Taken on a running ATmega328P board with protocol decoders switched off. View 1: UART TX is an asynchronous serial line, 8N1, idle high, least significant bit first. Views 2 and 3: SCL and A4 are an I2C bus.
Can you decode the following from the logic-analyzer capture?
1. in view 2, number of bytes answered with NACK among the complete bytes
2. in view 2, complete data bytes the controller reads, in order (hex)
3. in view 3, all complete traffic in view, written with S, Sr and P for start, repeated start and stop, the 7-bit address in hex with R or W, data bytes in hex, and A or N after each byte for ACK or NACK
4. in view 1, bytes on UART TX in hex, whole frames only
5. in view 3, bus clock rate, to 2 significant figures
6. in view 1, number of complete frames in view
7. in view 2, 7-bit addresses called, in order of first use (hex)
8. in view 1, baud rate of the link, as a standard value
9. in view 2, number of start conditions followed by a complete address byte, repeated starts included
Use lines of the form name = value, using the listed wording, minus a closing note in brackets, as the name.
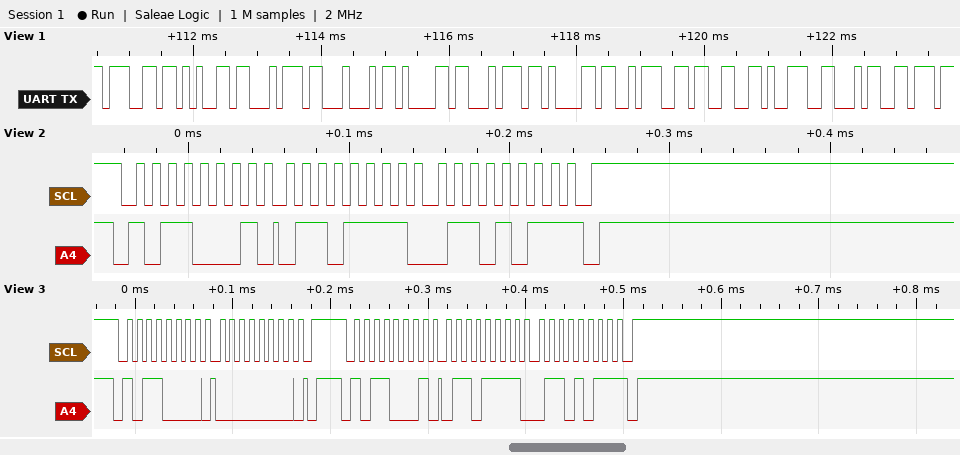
in view 2, number of bytes answered with NACK among the complete bytes = 1
in view 2, complete data bytes the controller reads, in order = 6F 6B
in view 3, all complete traffic in view, written with S, Sr and P for start, repeated start and stop, the 7-bit address in hex with R or W, data bytes in hex, and A or N after each byte for ACK or NACK = S 58W A 00 A P S 58R A 6F A 6B N P
in view 1, bytes on UART TX in hex, whole frames only = 0x67 0x65 0x74 0x44 0x61 0x74 0x61 0x3A 0x33 0x39 0x34
in view 3, bus clock rate, to 2 significant figures = 100 kHz
in view 1, number of complete frames in view = 11
in view 2, 7-bit addresses called, in order of first use = 0x58
in view 1, baud rate of the link, as a standard value = 9600 baud
in view 2, number of start conditions followed by a complete address byte, repeated starts included = 1
